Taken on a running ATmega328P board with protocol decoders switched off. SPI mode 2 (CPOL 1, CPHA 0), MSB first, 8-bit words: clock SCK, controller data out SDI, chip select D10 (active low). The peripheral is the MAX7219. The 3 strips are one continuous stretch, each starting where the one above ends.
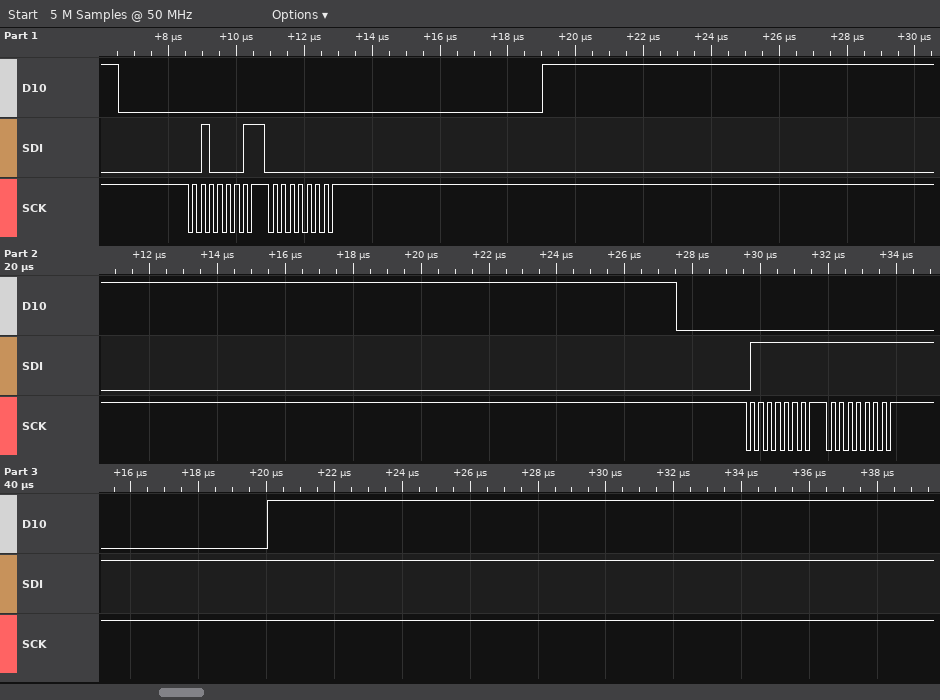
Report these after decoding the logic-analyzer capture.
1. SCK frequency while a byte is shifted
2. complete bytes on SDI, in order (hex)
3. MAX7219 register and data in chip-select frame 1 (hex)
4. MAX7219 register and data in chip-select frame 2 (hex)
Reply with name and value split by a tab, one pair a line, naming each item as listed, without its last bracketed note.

SCK frequency while a byte is shifted	4 MHz
complete bytes on SDI, in order	21 00 7F FF
MAX7219 register and data in chip-select frame 1	register 0x1, data 0x00
MAX7219 register and data in chip-select frame 2	register 0xF, data 0xFF
